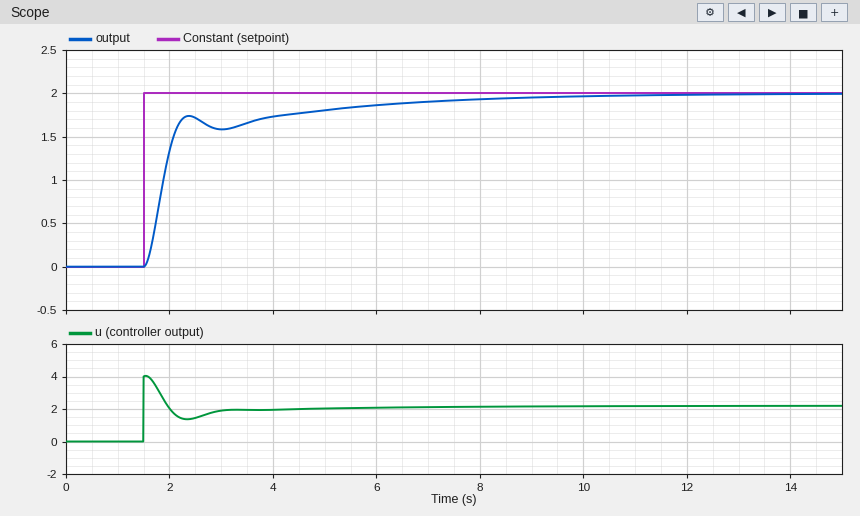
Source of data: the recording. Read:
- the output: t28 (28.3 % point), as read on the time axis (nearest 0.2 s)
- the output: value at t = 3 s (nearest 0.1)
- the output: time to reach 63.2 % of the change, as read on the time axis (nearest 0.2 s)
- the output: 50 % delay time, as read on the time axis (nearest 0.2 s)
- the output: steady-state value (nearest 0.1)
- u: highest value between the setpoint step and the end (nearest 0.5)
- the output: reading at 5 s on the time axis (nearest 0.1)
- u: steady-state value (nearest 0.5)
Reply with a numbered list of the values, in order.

1. 1.8 s
2. 1.6
3. 2.0 s
4. 1.8 s
5. 2.0
6. 4.0
7. 1.8
8. 2.0
